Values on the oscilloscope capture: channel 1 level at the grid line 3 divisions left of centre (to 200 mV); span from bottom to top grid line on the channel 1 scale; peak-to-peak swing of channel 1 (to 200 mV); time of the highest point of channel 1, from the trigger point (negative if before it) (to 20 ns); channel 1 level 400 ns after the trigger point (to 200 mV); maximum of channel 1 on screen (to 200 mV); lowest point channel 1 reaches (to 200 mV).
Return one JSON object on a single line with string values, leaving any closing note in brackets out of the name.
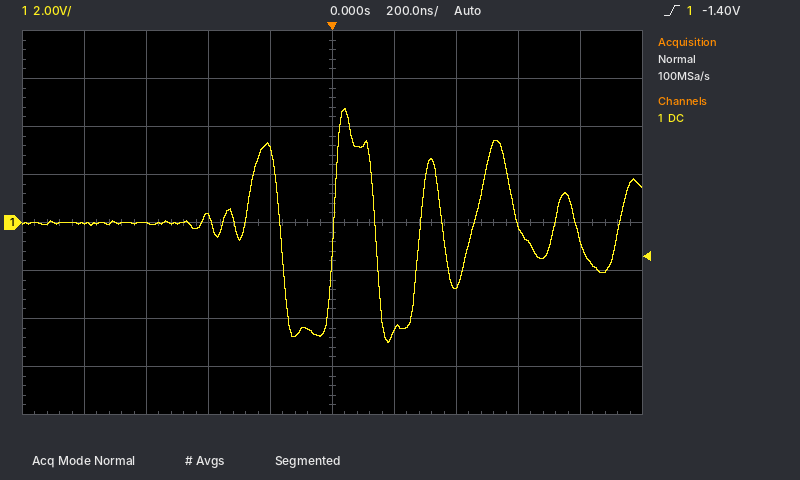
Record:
{"channel 1 level at the grid line 3 divisions left of centre": "0.0 V", "span from bottom to top grid line on the channel 1 scale": "16 V", "peak-to-peak swing of channel 1": "9.8 V", "time of the highest point of channel 1, from the trigger point (negative if before it)": "+40 ns", "channel 1 level 400 ns after the trigger point": "-2.6 V", "maximum of channel 1 on screen": "4.8 V", "lowest point channel 1 reaches": "-5.0 V"}
